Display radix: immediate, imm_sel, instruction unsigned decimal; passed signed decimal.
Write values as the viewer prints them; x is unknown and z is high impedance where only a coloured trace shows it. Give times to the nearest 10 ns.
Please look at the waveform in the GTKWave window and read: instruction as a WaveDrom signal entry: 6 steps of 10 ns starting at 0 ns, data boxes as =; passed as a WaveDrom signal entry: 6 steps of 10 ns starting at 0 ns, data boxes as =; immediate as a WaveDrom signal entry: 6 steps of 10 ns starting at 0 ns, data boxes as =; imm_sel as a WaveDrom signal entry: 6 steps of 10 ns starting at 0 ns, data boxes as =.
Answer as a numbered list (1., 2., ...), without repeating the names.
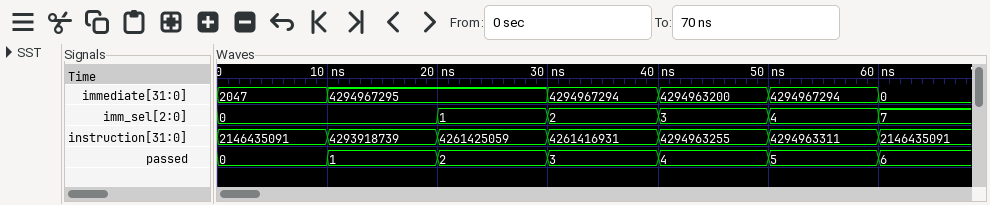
1. {name: 'instruction', wave: '======', data: '2146435091 4293918739 4261425059 4261416931 4294963255 4294963311'}
2. {name: 'passed', wave: '======', data: '0 1 2 3 4 5'}
3. {name: 'immediate', wave: '==.===', data: '2047 4294967295 4294967294 4294963200 4294967294'}
4. {name: 'imm_sel', wave: '=.====', data: '0 1 2 3 4'}
